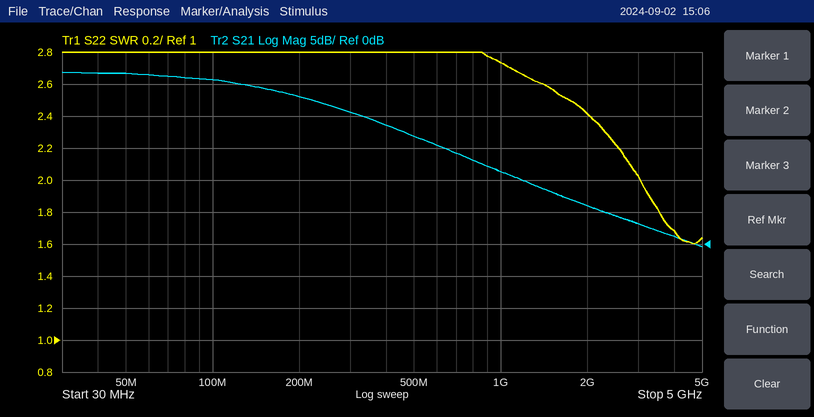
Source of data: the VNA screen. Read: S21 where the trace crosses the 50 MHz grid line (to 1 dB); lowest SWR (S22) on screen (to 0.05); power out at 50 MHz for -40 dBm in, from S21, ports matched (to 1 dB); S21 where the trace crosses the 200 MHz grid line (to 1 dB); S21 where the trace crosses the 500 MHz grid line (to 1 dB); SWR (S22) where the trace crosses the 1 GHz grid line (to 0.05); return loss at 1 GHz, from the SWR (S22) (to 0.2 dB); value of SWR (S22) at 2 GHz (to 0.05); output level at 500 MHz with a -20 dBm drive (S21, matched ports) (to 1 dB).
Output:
27 dB
1.60
-13 dBm
23 dB
17 dB
2.75
6.6 dB
2.40
-3 dBm
